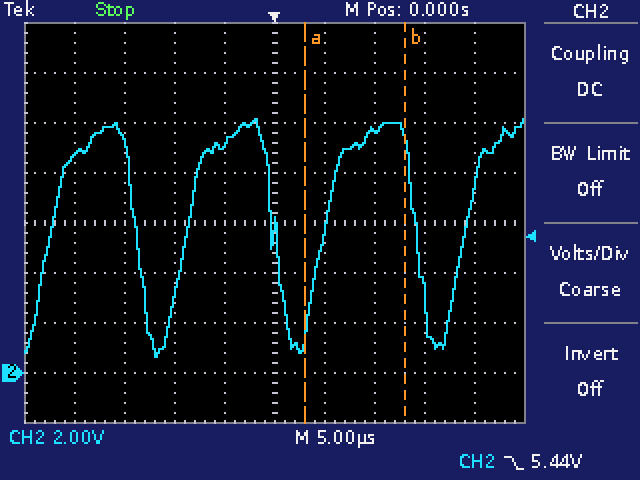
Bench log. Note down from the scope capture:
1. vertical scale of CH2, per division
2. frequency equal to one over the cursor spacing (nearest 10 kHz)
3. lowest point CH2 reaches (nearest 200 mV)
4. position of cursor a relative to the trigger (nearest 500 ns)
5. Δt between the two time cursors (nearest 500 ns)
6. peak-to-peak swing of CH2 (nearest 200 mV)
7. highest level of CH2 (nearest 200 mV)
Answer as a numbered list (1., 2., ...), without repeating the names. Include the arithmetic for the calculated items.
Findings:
1. 2 V
2. 1 / 10.0 µs ≈ 100 kHz
3. 600 mV
4. +3.0 µs
5. 10.0 µs
6. 10.2 V − (600 mV) = 9.6 V
7. 10.2 V
